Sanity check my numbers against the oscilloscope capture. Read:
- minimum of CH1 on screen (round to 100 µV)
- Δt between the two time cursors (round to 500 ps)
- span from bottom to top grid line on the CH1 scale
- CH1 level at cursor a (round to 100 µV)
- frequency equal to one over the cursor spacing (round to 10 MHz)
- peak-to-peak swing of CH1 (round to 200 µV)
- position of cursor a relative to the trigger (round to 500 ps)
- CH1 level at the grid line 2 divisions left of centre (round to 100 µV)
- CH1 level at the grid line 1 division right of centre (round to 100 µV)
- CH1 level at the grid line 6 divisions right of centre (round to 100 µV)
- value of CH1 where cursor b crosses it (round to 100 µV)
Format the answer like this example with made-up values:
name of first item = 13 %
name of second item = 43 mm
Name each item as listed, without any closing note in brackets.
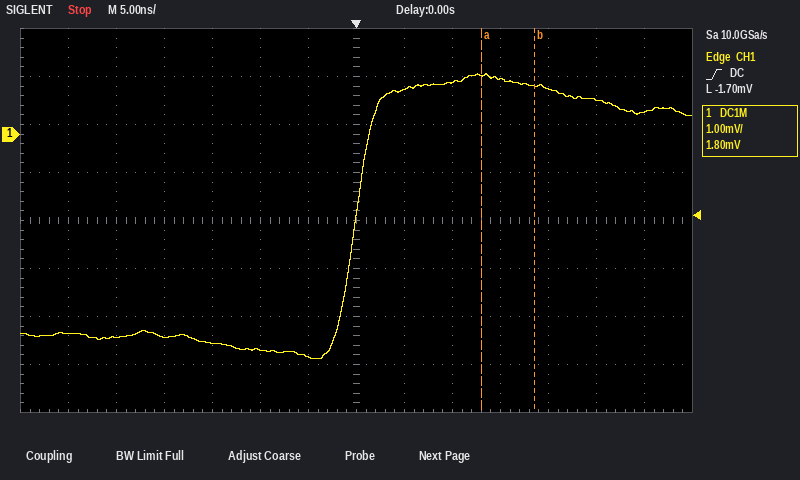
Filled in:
minimum of CH1 on screen = -4.7 mV
Δt between the two time cursors = 5.5 ns
span from bottom to top grid line on the CH1 scale = 8 mV
CH1 level at cursor a = 1.2 mV
frequency equal to one over the cursor spacing = 180 MHz
peak-to-peak swing of CH1 = 6.0 mV
position of cursor a relative to the trigger = +13.0 ns
CH1 level at the grid line 2 divisions left of centre = -4.5 mV
CH1 level at the grid line 1 division right of centre = 900 µV
CH1 level at the grid line 6 divisions right of centre = 500 µV
value of CH1 where cursor b crosses it = 1.0 mV
